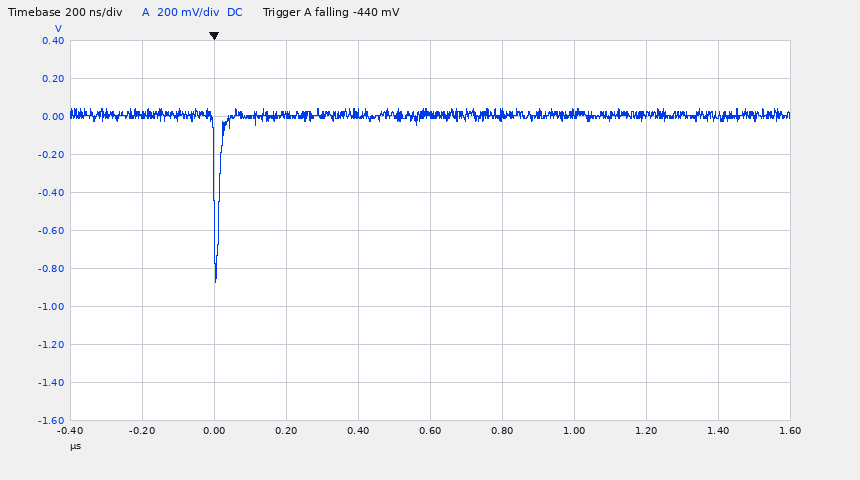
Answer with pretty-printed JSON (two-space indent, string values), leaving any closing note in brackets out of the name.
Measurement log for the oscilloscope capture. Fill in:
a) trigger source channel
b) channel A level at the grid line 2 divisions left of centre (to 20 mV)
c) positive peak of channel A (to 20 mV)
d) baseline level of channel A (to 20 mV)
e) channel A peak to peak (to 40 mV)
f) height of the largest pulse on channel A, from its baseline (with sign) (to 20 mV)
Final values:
{
  "trigger source channel": "channel A",
  "channel A level at the grid line 2 divisions left of centre": "0 mV",
  "positive peak of channel A": "40 mV",
  "baseline level of channel A": "0 mV",
  "channel A peak to peak": "920 mV",
  "height of the largest pulse on channel A, from its baseline (with sign)": "-880 mV"
}
